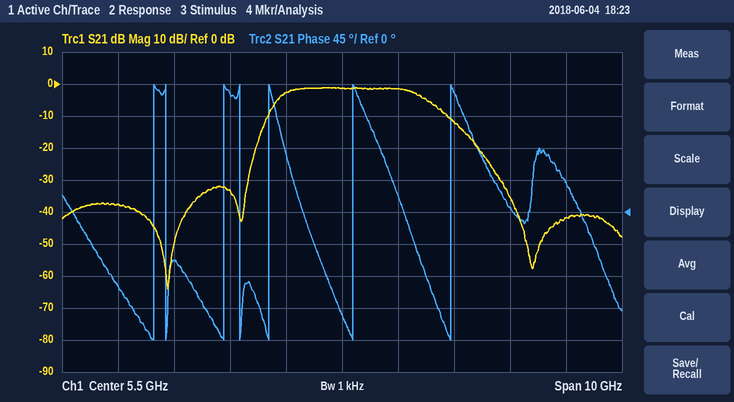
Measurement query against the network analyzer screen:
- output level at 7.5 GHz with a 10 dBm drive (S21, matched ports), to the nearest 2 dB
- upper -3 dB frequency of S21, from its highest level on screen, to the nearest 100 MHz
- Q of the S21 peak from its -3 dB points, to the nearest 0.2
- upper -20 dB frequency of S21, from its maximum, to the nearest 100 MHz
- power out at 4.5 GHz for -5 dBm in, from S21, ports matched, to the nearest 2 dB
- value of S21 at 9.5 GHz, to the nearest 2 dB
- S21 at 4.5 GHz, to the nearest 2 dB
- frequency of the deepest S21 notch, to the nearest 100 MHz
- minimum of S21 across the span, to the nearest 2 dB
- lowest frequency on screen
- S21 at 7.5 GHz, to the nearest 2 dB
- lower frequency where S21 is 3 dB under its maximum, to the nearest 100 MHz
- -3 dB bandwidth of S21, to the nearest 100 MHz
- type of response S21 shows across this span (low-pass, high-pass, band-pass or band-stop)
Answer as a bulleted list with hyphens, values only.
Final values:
- -2 dBm
- 6.9 GHz
- 2.2
- 8.0 GHz
- -8 dBm
- -42 dB
- -2 dB
- 2.4 GHz
- -64 dB
- 500 MHz
- -12 dB
- 4.4 GHz
- 2.5 GHz
- band-pass
